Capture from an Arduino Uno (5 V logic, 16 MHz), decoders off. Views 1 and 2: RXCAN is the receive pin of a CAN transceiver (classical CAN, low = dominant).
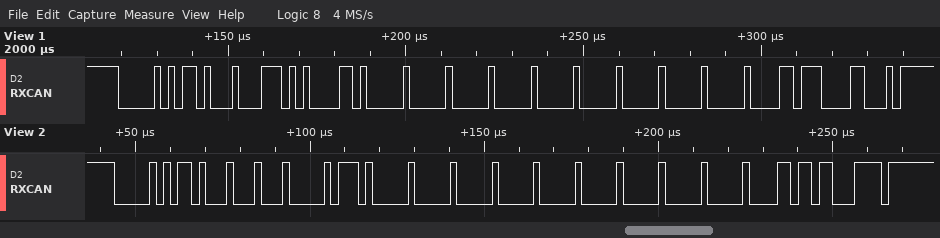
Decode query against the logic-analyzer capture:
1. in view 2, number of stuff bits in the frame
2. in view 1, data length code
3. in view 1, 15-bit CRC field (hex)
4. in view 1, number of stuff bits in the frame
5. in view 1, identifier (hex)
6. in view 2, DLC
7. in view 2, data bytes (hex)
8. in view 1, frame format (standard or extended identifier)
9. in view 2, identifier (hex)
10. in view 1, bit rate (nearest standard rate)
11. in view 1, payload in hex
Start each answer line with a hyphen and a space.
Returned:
- 11
- 8
- 0x6E18
- 10
- 0x02D
- 8
- 88 1D 00 00 00 00 00 00
- standard
- 0x02D
- 500 kbit/s
- EA 1A 00 00 00 00 00 00
